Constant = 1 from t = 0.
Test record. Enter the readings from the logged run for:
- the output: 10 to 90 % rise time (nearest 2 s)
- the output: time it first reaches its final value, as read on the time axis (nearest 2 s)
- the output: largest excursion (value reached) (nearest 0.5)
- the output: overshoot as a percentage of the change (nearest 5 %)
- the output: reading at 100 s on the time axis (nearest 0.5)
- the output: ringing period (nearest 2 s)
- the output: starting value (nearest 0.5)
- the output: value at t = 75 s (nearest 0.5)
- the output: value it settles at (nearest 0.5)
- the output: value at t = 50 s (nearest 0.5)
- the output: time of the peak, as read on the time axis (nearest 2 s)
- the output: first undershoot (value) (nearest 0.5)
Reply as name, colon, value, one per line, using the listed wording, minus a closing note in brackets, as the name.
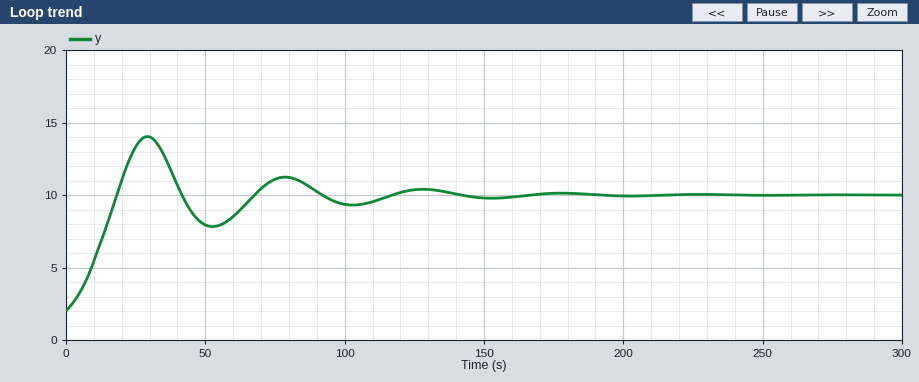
the output: 10 to 90 % rise time: 14 s
the output: time it first reaches its final value, as read on the time axis: 18 s
the output: largest excursion (value reached): 14.0
the output: overshoot as a percentage of the change: 50 %
the output: reading at 100 s on the time axis: 9.5
the output: ringing period: 50 s
the output: starting value: 2.0
the output: value at t = 75 s: 11.0
the output: value it settles at: 10.0
the output: value at t = 50 s: 8.0
the output: time of the peak, as read on the time axis: 30 s
the output: first undershoot (value): 8.0
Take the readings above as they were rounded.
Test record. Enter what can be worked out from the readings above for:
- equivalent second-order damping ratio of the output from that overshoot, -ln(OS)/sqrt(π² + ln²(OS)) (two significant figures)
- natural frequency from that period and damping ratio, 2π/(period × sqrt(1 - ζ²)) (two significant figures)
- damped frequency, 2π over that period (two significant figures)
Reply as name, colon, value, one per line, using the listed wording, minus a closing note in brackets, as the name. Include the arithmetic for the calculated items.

equivalent second-order damping ratio of the output from that overshoot, -ln(OS)/sqrt(π² + ln²(OS)): ln(0.5) = -0.693; 0.693 / sqrt(9.870 + 0.480) = 0.22
natural frequency from that period and damping ratio, 2π/(period × sqrt(1 - ζ²)): 2π / (50 × sqrt(1 - 0.22²)) = 0.13 rad/s
damped frequency, 2π over that period: 2π / 50 = 0.13 rad/s
